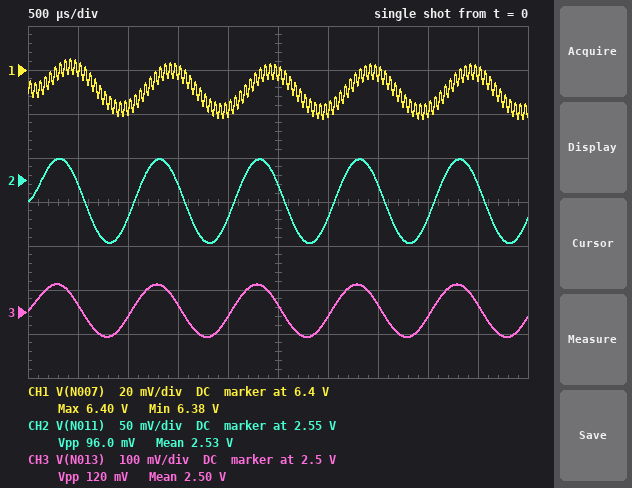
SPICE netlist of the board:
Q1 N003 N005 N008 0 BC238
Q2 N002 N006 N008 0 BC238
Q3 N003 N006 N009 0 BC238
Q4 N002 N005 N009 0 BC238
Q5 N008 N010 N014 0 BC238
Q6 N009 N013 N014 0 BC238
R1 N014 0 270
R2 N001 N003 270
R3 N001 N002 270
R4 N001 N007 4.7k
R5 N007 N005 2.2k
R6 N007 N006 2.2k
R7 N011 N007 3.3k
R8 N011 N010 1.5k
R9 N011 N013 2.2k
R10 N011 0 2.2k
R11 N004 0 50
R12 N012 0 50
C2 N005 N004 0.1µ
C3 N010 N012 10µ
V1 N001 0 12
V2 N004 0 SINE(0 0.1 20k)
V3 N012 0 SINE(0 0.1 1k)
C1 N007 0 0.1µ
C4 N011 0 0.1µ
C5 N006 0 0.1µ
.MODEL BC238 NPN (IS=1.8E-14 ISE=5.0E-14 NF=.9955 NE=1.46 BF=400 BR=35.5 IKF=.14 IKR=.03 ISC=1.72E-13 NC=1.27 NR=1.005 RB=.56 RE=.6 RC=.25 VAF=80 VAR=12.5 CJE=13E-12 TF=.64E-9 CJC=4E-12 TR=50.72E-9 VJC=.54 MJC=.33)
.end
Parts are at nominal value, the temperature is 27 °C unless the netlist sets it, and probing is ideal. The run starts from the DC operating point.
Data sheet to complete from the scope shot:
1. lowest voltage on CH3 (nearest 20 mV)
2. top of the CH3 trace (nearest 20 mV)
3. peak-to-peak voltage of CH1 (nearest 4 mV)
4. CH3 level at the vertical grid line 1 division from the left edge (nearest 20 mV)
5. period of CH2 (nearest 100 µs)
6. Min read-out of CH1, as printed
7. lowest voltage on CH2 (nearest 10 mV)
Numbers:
2.44 V
2.56 V
28 mV
2.52 V
1.0 ms
6.38 V
2.48 V
